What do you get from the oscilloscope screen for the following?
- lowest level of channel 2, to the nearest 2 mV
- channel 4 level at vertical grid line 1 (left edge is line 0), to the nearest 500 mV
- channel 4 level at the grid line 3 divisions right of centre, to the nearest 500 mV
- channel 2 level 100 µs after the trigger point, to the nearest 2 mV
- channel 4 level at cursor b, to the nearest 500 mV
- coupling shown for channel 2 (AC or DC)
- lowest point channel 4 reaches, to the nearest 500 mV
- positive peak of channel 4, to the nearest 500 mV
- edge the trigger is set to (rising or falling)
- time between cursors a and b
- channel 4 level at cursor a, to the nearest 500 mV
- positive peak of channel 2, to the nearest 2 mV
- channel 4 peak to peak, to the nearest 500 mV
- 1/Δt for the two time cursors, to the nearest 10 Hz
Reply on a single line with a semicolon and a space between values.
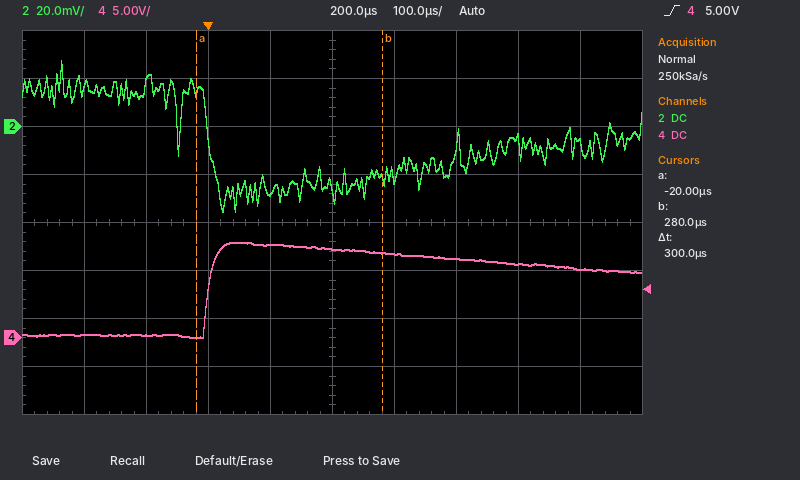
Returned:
-36 mV; 500 mV; 7.5 V; -28 mV; 9.0 V; DC; 0.0 V; 10.0 V; rising; 300 µs; 0.0 V; 28 mV; 10.0 V; 3.33 kHz
